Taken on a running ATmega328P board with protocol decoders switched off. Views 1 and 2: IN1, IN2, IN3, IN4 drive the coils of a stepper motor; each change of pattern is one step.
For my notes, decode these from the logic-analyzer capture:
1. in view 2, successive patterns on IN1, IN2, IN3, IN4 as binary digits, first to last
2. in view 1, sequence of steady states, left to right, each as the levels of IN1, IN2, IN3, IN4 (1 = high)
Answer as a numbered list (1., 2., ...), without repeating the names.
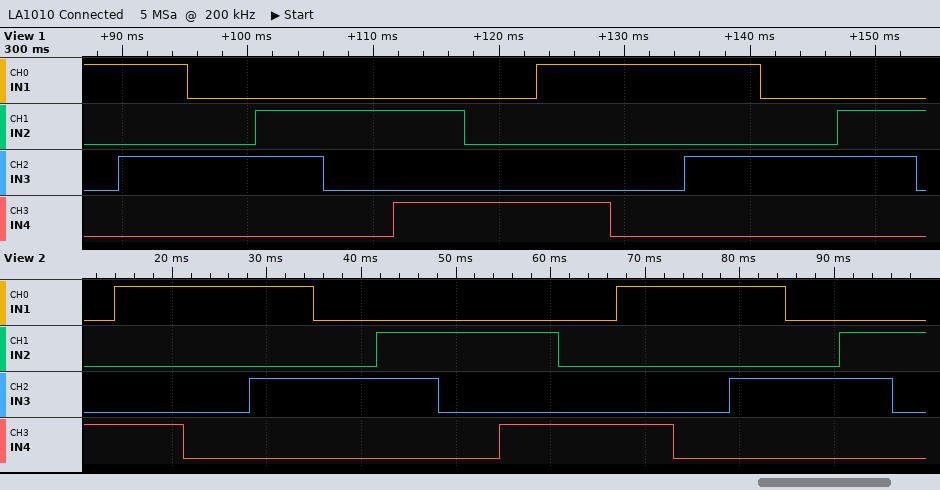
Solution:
1. 0001 1001 1000 1010 0010 0110 0100 0101 0001 1001 1000 1010 0010 0110 0100
2. 1000 1010 0010 0110 0100 0101 0001 1001 1000 1010 0010 0110 0100
